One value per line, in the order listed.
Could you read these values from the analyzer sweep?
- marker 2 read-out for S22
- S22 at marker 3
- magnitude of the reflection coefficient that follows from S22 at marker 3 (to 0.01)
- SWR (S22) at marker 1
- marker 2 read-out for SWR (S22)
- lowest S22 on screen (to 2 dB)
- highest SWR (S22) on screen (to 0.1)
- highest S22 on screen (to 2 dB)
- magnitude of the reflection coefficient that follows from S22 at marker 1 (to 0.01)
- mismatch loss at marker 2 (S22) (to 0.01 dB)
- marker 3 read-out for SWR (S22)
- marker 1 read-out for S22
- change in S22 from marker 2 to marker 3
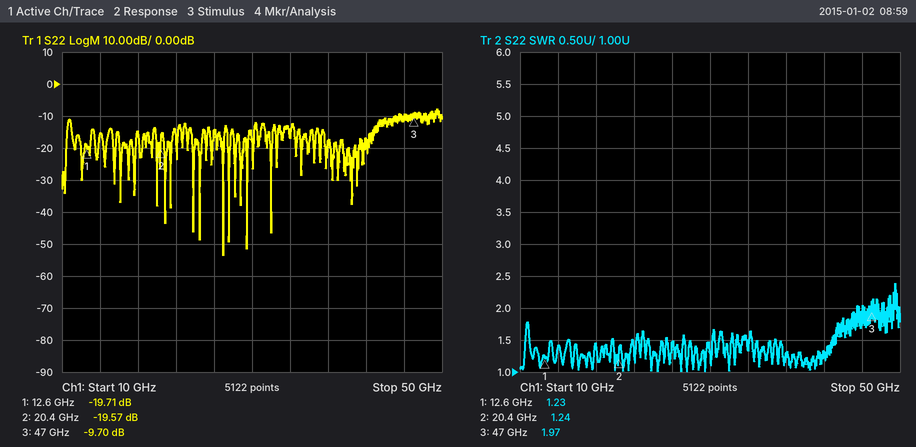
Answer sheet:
-19.57 dB
-9.70 dB
0.33
1.23
1.24
-54 dB
2.4
-8 dB
0.10
0.05 dB
1.97
-19.71 dB
9.87 dB
